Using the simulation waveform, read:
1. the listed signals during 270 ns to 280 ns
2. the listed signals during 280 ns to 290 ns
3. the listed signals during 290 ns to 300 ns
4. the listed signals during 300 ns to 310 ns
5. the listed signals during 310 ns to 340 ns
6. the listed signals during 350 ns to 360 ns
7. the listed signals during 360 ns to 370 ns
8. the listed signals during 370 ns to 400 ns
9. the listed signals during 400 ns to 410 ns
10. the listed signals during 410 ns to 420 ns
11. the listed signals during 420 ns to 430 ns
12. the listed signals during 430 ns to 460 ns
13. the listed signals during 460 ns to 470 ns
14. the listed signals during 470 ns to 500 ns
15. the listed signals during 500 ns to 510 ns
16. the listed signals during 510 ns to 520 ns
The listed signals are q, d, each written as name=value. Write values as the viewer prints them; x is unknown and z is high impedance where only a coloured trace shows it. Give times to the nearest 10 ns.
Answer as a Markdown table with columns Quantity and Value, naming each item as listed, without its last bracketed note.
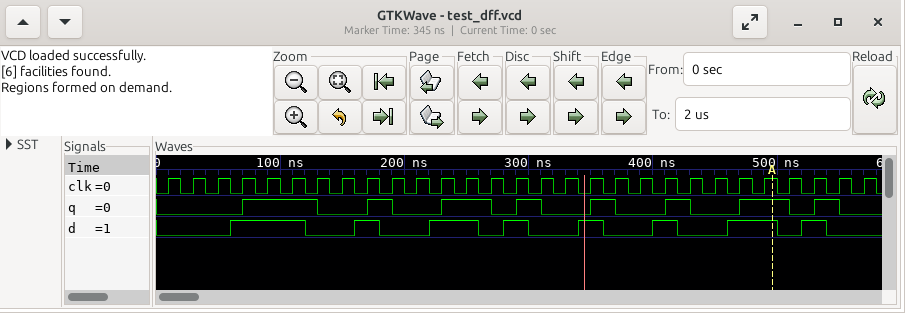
| Quantity | Value |
|---|---|
| the listed signals during 270 ns to 280 ns | q=0, d=0 |
| the listed signals during 280 ns to 290 ns | q=0, d=1 |
| the listed signals during 290 ns to 300 ns | q=1, d=1 |
| the listed signals during 300 ns to 310 ns | q=1, d=0 |
| the listed signals during 310 ns to 340 ns | q=0, d=0 |
| the listed signals during 350 ns to 360 ns | q=1, d=1 |
| the listed signals during 360 ns to 370 ns | q=1, d=0 |
| the listed signals during 370 ns to 400 ns | q=0, d=0 |
| the listed signals during 400 ns to 410 ns | q=0, d=1 |
| the listed signals during 410 ns to 420 ns | q=1, d=1 |
| the listed signals during 420 ns to 430 ns | q=1, d=0 |
| the listed signals during 430 ns to 460 ns | q=0, d=0 |
| the listed signals during 460 ns to 470 ns | q=0, d=1 |
| the listed signals during 470 ns to 500 ns | q=1, d=1 |
| the listed signals during 500 ns to 510 ns | q=1, d=0 |
| the listed signals during 510 ns to 520 ns | q=0, d=0 |
